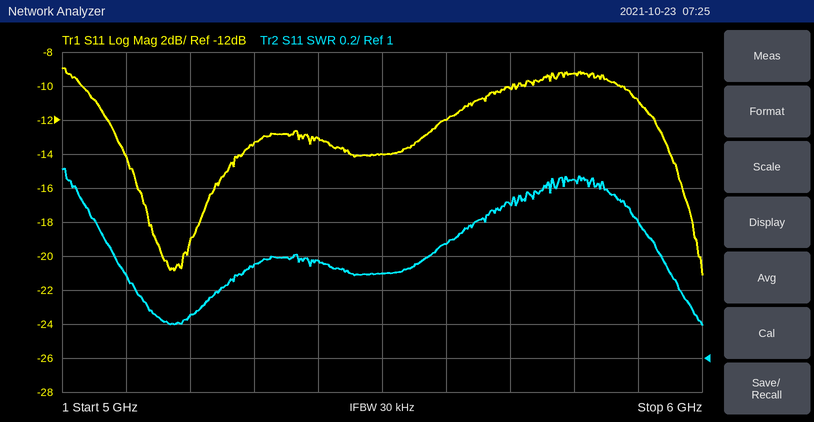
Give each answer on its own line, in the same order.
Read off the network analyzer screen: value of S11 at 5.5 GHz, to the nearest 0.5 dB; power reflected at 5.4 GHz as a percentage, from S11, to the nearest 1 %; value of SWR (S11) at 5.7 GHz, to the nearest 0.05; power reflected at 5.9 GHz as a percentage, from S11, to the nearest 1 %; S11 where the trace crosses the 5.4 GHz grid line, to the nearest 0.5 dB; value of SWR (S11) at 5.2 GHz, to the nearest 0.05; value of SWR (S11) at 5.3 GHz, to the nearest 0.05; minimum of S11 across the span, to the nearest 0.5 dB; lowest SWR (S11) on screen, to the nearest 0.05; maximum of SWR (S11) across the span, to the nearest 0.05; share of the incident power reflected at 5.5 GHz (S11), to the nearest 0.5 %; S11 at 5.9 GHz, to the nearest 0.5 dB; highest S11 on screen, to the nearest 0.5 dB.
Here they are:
-14.0 dB
5 %
1.90
8 %
-13.0 dB
1.25
1.55
-21.0 dB
1.20
2.10
4.0 %
-11.0 dB
-9.0 dB
